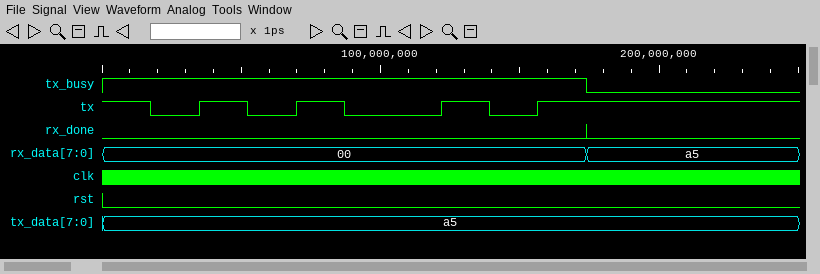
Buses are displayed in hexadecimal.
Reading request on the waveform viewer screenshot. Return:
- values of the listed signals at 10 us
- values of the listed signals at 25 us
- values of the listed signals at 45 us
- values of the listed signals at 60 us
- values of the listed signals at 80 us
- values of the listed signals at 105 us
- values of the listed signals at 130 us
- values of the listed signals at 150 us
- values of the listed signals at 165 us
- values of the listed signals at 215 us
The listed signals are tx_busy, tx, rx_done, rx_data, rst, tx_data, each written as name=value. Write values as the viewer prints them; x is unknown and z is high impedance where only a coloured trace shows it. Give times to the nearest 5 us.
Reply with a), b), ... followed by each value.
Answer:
a) tx_busy=1, tx=1, rx_done=0, rx_data=00, rst=0, tx_data=a5
b) tx_busy=1, tx=0, rx_done=0, rx_data=00, rst=0, tx_data=a5
c) tx_busy=1, tx=1, rx_done=0, rx_data=00, rst=0, tx_data=a5
d) tx_busy=1, tx=0, rx_done=0, rx_data=00, rst=0, tx_data=a5
e) tx_busy=1, tx=1, rx_done=0, rx_data=00, rst=0, tx_data=a5
f) tx_busy=1, tx=0, rx_done=0, rx_data=00, rst=0, tx_data=a5
g) tx_busy=1, tx=1, rx_done=0, rx_data=00, rst=0, tx_data=a5
h) tx_busy=1, tx=0, rx_done=0, rx_data=00, rst=0, tx_data=a5
i) tx_busy=1, tx=1, rx_done=0, rx_data=00, rst=0, tx_data=a5
j) tx_busy=0, tx=1, rx_done=0, rx_data=a5, rst=0, tx_data=a5
